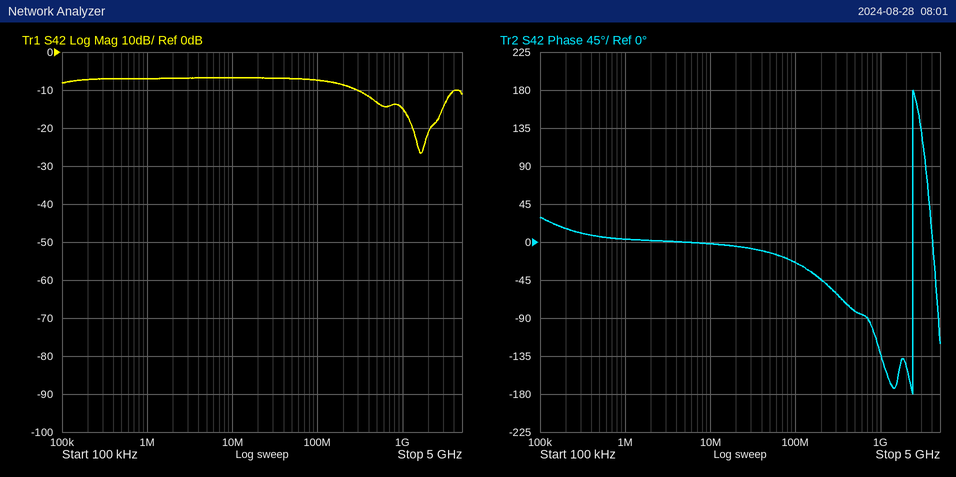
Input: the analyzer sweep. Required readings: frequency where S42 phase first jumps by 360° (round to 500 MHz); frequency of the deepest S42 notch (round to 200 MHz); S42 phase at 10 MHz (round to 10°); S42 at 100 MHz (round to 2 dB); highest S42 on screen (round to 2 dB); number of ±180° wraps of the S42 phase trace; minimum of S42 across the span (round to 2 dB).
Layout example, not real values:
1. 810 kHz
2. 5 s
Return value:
1. 2.5 GHz
2. 1.6 GHz
3. 0°
4. -8 dB
5. -6 dB
6. 1
7. -26 dB
